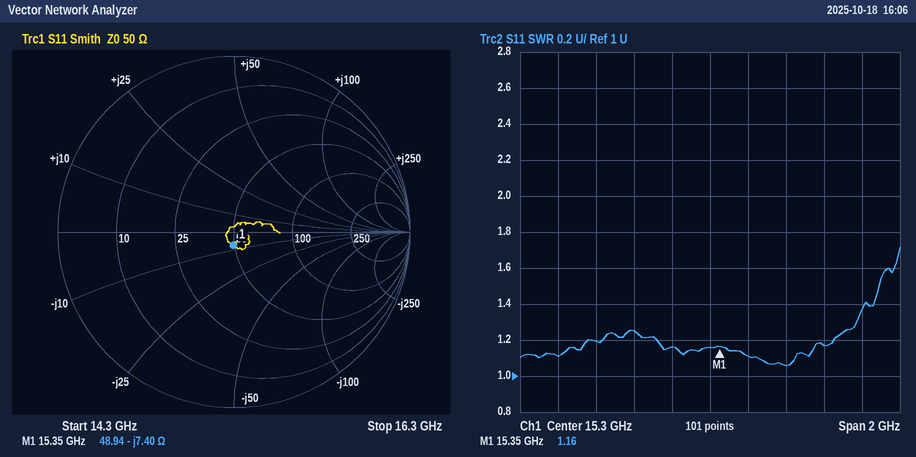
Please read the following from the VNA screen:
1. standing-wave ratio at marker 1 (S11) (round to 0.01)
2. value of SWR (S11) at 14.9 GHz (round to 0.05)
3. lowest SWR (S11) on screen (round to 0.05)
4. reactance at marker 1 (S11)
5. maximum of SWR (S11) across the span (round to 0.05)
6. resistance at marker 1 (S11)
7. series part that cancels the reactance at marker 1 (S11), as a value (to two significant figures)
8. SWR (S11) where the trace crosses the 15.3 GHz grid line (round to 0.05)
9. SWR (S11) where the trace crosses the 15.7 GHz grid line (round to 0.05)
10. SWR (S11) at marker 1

1.16
1.25
1.05
-7.40 Ω
1.70
48.94 Ω
77 pH
1.15
1.05
1.16
